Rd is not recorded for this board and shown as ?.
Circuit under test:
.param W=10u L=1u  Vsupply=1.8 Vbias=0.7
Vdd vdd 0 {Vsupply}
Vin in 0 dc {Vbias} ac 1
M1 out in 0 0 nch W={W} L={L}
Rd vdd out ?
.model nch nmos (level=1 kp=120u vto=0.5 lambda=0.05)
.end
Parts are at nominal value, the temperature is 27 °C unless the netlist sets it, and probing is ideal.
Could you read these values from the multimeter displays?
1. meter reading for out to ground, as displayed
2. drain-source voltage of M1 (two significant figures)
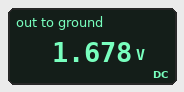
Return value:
1.678 V
1.7 V
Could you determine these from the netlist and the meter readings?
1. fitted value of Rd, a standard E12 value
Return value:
4.7 kΩ
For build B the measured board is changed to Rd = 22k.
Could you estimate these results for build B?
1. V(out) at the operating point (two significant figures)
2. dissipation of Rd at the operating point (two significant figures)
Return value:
1.2 V
14 µW
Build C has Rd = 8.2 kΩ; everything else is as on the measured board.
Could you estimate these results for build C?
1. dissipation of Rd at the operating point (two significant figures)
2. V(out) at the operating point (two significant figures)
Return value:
5.5 µW
1.6 V
